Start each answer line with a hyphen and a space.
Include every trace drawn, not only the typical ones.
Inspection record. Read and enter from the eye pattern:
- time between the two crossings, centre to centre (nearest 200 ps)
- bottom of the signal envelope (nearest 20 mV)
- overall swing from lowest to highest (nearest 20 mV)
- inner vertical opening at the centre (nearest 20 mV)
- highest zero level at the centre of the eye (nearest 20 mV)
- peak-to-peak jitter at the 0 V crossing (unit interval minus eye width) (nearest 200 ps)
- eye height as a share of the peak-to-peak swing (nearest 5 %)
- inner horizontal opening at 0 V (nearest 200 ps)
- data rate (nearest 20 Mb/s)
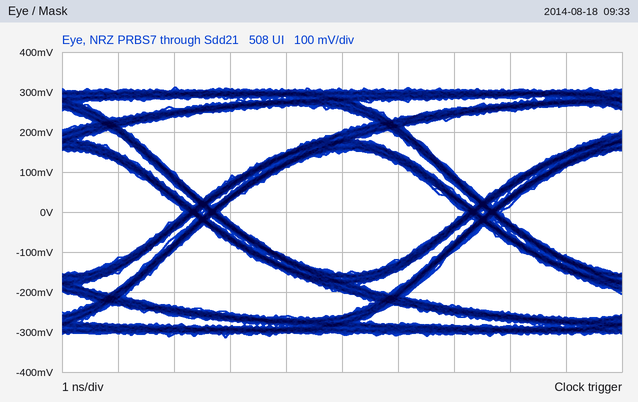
- 5.0 ns
- -320 mV
- 620 mV
- 300 mV
- -160 mV
- 600 ps
- 50 %
- 4.4 ns
- 200 Mb/s
